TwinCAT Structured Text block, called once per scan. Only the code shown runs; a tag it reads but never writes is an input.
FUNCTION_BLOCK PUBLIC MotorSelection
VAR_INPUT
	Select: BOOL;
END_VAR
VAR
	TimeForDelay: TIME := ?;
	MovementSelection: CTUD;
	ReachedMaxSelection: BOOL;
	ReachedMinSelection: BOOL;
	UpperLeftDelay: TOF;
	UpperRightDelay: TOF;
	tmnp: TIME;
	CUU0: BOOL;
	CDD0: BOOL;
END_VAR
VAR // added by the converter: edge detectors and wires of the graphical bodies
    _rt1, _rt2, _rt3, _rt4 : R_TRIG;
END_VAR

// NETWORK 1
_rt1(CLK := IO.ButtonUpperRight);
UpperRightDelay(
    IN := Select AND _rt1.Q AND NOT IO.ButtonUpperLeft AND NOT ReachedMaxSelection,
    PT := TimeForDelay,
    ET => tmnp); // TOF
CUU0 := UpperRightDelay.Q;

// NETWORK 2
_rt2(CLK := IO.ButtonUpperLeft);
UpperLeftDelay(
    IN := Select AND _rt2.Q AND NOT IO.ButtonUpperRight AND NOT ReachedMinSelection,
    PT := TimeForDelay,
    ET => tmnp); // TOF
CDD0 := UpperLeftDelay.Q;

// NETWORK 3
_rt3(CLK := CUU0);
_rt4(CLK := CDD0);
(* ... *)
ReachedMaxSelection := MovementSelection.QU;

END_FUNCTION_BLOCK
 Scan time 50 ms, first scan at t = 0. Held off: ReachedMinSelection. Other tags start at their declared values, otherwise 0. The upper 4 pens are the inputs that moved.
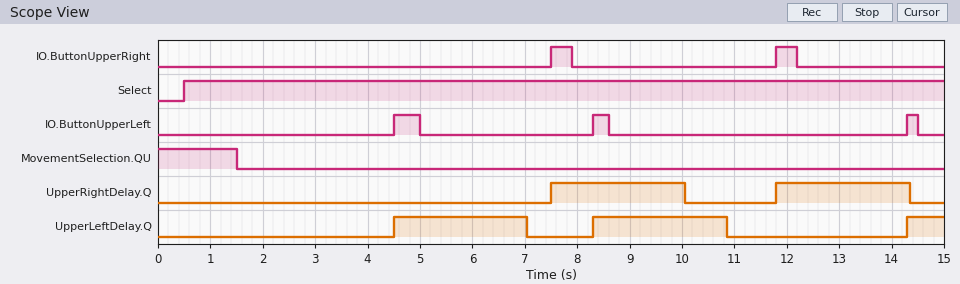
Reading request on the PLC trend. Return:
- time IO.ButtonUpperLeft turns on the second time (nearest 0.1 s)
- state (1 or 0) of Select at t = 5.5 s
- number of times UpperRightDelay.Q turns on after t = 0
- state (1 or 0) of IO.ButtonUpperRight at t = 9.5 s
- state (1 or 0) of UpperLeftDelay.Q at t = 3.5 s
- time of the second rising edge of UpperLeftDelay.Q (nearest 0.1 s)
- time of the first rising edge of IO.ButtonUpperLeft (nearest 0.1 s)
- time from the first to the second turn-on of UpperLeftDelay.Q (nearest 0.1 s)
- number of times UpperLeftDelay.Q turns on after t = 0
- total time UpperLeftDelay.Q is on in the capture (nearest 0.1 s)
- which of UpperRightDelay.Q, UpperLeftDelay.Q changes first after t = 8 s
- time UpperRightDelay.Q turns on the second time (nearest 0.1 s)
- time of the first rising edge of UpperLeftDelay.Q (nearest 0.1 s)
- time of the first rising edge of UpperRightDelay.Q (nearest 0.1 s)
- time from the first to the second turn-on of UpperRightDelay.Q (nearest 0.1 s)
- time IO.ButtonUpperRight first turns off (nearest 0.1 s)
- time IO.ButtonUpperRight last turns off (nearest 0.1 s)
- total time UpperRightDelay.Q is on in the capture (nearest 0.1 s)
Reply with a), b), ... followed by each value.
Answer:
a) 8.3 s
b) 1
c) 2
d) 0
e) 0
f) 8.3 s
g) 4.5 s
h) 3.8 s
i) 3
j) 5.8 s
k) UpperLeftDelay.Q
l) 11.8 s
m) 4.5 s
n) 7.5 s
o) 4.3 s
p) 7.9 s
q) 12.2 s
r) 5.1 s
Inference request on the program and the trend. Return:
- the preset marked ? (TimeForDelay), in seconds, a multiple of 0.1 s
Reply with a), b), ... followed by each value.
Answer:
a) 2.5 s
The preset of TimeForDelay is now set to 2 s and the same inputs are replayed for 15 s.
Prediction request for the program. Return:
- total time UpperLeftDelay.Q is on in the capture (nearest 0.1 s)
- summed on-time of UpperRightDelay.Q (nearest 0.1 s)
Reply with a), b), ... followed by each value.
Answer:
a) 4.8 s
b) 4.1 s
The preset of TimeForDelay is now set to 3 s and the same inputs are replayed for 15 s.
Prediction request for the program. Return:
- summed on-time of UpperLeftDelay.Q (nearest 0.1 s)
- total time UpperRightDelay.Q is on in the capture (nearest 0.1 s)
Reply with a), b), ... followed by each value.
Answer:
a) 6.8 s
b) 6.1 s
